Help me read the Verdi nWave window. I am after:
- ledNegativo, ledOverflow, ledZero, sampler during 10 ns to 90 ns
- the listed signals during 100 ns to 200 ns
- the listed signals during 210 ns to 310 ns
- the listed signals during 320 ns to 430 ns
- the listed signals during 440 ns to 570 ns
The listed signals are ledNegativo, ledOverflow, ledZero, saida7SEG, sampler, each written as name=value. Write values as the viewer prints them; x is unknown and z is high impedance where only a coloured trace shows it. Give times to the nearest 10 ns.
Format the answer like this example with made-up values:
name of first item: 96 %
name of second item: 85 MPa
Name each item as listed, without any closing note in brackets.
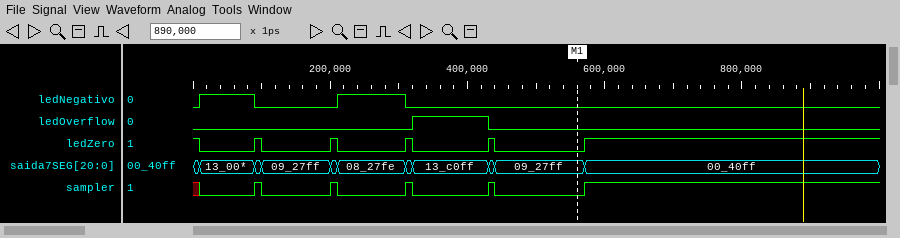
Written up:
ledNegativo, ledOverflow, ledZero, sampler during 10 ns to 90 ns: ledNegativo=1, ledOverflow=0, ledZero=0, sampler=0
the listed signals during 100 ns to 200 ns: ledNegativo=0, ledOverflow=0, ledZero=0, saida7SEG=09_27ff, sampler=0
the listed signals during 210 ns to 310 ns: ledNegativo=1, ledOverflow=0, ledZero=0, saida7SEG=08_27fe, sampler=0
the listed signals during 320 ns to 430 ns: ledNegativo=0, ledOverflow=1, ledZero=0, saida7SEG=13_c0ff, sampler=0
the listed signals during 440 ns to 570 ns: ledNegativo=0, ledOverflow=0, ledZero=0, saida7SEG=09_27ff, sampler=0
